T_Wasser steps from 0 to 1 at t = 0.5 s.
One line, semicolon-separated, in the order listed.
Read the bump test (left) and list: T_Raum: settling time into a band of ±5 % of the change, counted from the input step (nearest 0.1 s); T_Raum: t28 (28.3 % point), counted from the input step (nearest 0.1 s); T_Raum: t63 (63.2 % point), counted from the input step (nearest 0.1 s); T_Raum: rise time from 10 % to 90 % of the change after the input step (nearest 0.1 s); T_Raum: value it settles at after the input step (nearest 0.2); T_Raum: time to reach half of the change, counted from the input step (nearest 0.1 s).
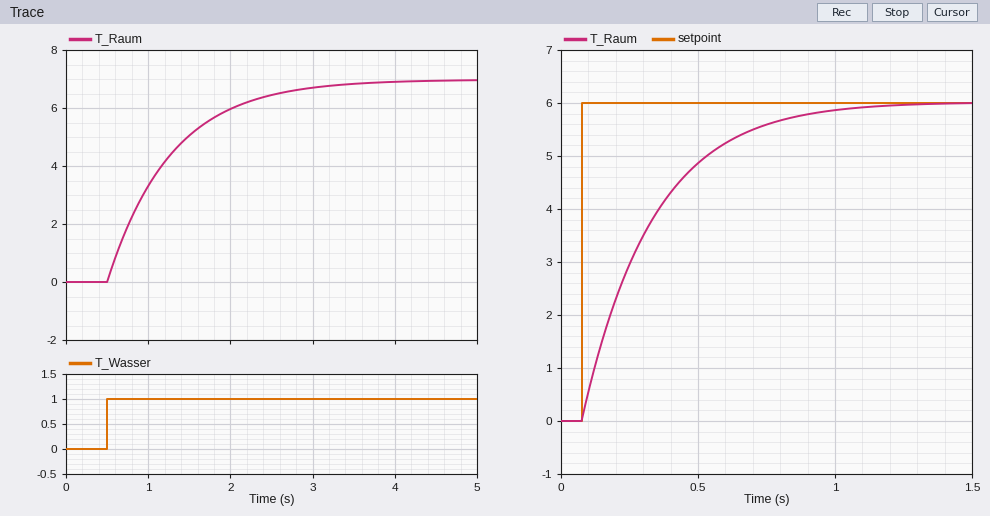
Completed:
2.3 s; 0.3 s; 0.8 s; 1.7 s; 7.0; 0.5 s
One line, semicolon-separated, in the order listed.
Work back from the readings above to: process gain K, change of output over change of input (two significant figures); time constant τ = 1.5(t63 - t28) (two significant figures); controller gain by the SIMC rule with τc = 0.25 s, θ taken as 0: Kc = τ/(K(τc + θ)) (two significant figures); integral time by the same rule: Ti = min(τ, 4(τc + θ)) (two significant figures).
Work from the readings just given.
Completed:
7.0; 0.75 s; 0.43; 0.75 s
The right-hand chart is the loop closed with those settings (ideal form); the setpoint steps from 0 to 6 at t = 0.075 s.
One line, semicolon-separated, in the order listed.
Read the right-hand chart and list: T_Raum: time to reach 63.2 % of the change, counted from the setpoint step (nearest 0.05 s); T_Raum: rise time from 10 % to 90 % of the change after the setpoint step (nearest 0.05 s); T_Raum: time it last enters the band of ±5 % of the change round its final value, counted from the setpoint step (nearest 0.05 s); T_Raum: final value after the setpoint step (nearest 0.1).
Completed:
0.25 s; 0.55 s; 0.75 s; 6.0
